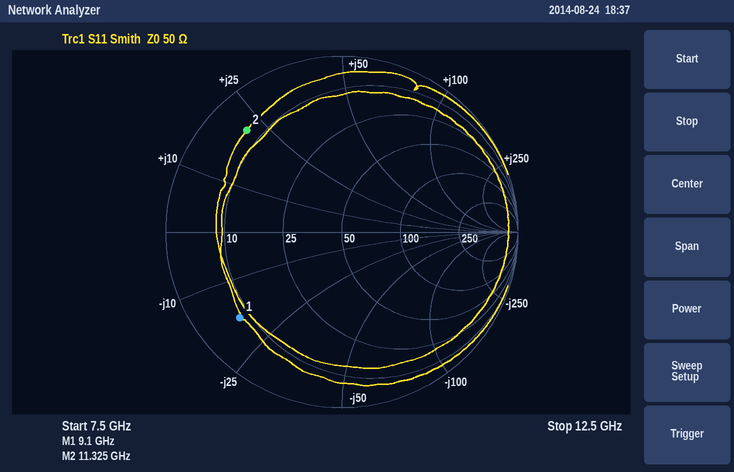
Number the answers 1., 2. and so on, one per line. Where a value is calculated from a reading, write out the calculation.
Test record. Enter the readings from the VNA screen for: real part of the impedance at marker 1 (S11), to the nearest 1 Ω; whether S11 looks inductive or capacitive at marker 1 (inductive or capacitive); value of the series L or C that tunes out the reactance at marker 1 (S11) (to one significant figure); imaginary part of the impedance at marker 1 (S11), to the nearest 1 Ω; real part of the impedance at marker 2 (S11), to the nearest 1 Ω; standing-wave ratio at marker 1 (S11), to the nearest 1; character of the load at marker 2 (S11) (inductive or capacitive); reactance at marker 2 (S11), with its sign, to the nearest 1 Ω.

1. 8 Ω
2. capacitive
3. L = 18 Ω/(2π × 9.1 GHz) ≈ 315 pH, so 300 pH to one significant figure
4. -18 Ω
5. 7 Ω
6. 7
7. inductive
8. +21 Ω
